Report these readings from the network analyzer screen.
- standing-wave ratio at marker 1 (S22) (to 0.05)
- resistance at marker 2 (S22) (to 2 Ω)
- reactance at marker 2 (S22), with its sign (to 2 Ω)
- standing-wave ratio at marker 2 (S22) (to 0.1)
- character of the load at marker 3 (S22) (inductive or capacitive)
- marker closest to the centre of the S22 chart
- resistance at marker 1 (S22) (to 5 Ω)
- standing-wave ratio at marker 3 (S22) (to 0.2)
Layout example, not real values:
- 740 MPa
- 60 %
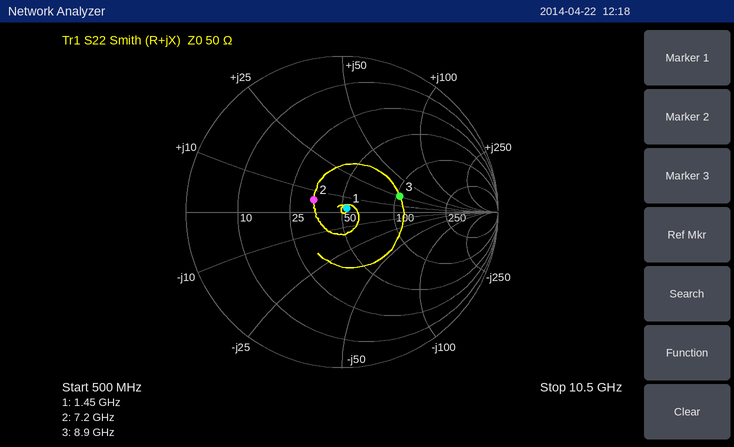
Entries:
- 1.10
- 34 Ω
- +6 Ω
- 1.5
- inductive
- marker 1
- 55 Ω
- 2.2
